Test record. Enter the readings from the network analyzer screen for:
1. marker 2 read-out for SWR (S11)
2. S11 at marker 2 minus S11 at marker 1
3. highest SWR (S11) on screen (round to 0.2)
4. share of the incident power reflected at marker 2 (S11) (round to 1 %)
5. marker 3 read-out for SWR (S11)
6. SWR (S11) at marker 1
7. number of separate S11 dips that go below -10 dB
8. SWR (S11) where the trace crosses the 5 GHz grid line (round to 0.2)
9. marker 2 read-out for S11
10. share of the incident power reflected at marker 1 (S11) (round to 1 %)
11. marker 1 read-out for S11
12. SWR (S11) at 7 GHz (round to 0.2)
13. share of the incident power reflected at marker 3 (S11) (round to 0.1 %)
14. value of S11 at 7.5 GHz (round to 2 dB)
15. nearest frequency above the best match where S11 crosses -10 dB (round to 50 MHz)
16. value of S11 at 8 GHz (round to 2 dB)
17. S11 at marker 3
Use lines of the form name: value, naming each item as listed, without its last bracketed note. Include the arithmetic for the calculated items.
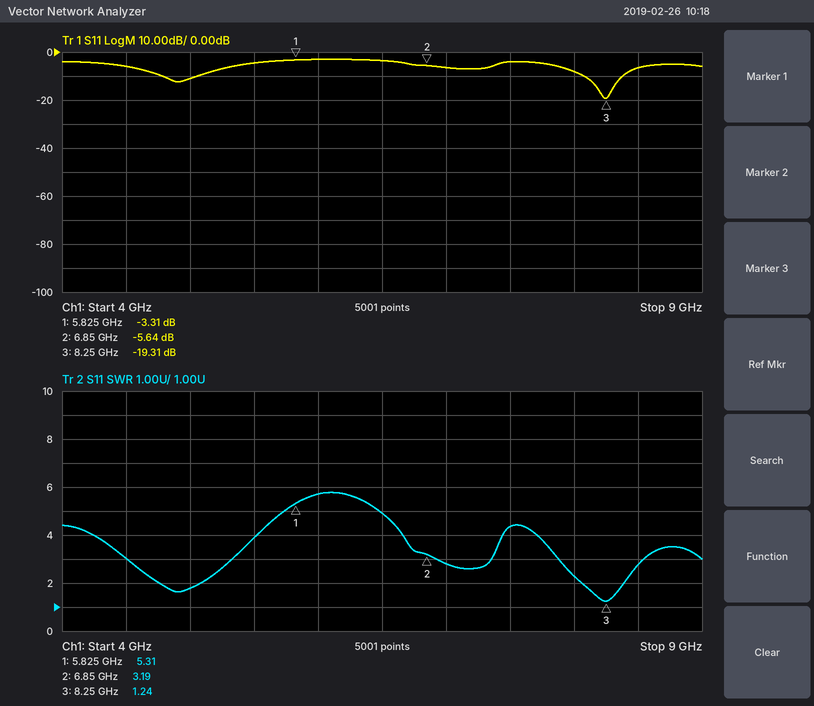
marker 2 read-out for SWR: 3.19
S11 at marker 2 minus S11 at marker 1: -5.64 − (-3.31) = -2.33 dB
highest SWR (S11) on screen: 5.8
share of the incident power reflected at marker 2 (S11): 10^(-5.64/10) ≈ 27 %
marker 3 read-out for SWR: 1.24
SWR (S11) at marker 1: 5.31
number of separate S11 dips that go below -10 dB: 2
SWR (S11) where the trace crosses the 5 GHz grid line: 1.8
marker 2 read-out for S11: -5.64 dB
share of the incident power reflected at marker 1 (S11): 10^(-3.31/10) ≈ 47 %
marker 1 read-out for S11: -3.31 dB
SWR (S11) at 7 GHz: 2.8
share of the incident power reflected at marker 3 (S11): 10^(-19.31/10) ≈ 1.2 %
value of S11 at 7.5 GHz: -4 dB
nearest frequency above the best match where S11 crosses -10 dB: 8.40 GHz
value of S11 at 8 GHz: -8 dB
S11 at marker 3: -19.31 dB
